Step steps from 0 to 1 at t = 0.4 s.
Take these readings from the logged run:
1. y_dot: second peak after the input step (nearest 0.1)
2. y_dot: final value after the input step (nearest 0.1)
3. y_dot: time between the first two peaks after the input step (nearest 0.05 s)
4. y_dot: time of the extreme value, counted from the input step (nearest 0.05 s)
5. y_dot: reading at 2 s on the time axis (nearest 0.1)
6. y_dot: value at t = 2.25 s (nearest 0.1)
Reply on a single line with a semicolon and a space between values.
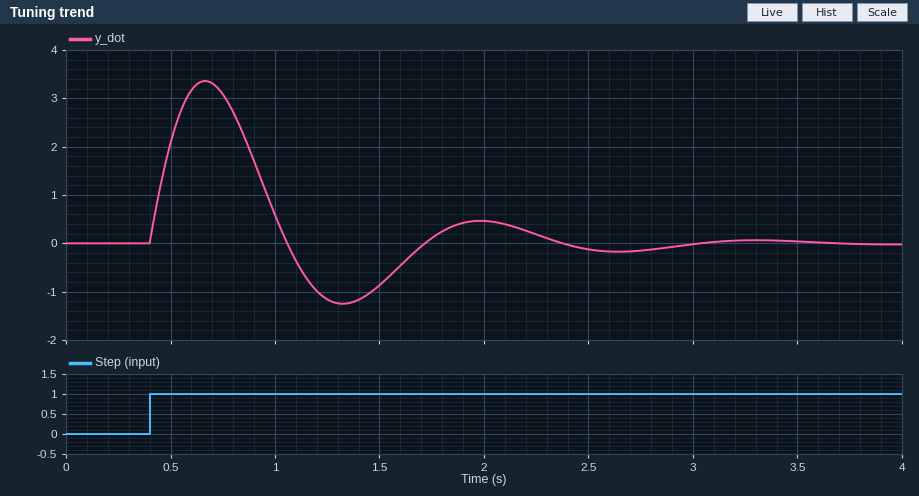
0.5; 0.0; 1.30 s; 0.25 s; 0.5; 0.2
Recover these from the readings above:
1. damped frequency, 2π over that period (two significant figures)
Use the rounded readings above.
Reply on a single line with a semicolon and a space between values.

4.8 rad/s
